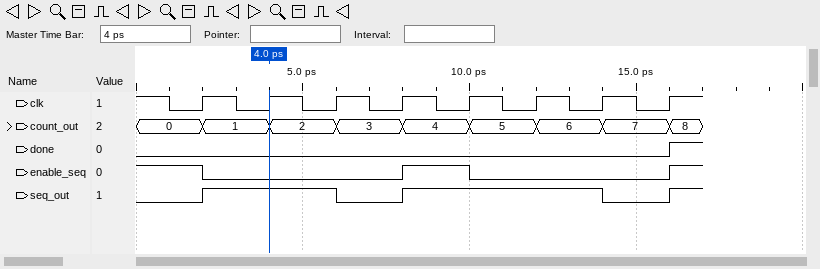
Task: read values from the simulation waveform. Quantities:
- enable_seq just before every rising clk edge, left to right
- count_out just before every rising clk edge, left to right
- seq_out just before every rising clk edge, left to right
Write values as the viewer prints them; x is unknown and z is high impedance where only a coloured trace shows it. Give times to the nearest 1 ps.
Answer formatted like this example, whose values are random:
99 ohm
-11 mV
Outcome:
1 0 0 0 1 0 0 0
0, 1, 2, 3, 4, 5, 6, 7
0 1 1 0 1 1 1 0
